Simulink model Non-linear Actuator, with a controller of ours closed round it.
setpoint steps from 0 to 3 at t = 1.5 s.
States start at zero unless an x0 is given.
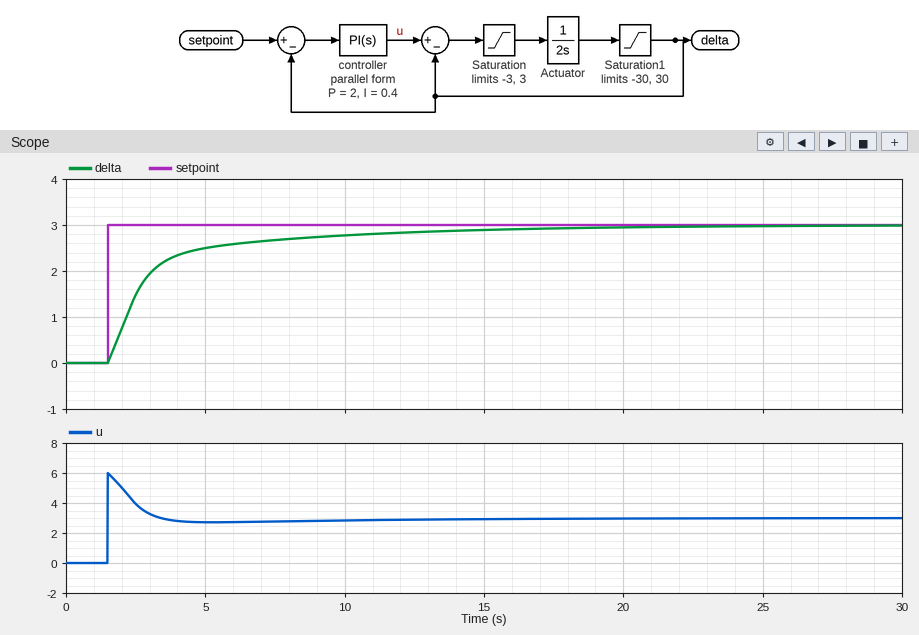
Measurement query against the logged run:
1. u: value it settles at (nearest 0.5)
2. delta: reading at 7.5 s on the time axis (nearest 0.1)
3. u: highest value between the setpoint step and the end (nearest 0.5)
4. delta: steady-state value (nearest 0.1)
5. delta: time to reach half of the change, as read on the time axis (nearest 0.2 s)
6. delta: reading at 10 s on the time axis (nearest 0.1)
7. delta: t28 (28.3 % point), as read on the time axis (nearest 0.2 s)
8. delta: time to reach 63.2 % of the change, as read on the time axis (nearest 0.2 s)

3.0
2.7
6.0
3.0
2.6 s
2.8
2.0 s
3.0 s
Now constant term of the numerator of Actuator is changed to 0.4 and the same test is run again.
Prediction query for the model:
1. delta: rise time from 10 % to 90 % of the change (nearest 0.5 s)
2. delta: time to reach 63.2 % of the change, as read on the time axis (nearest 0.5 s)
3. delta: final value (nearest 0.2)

5.0 s
4.5 s
3.0
